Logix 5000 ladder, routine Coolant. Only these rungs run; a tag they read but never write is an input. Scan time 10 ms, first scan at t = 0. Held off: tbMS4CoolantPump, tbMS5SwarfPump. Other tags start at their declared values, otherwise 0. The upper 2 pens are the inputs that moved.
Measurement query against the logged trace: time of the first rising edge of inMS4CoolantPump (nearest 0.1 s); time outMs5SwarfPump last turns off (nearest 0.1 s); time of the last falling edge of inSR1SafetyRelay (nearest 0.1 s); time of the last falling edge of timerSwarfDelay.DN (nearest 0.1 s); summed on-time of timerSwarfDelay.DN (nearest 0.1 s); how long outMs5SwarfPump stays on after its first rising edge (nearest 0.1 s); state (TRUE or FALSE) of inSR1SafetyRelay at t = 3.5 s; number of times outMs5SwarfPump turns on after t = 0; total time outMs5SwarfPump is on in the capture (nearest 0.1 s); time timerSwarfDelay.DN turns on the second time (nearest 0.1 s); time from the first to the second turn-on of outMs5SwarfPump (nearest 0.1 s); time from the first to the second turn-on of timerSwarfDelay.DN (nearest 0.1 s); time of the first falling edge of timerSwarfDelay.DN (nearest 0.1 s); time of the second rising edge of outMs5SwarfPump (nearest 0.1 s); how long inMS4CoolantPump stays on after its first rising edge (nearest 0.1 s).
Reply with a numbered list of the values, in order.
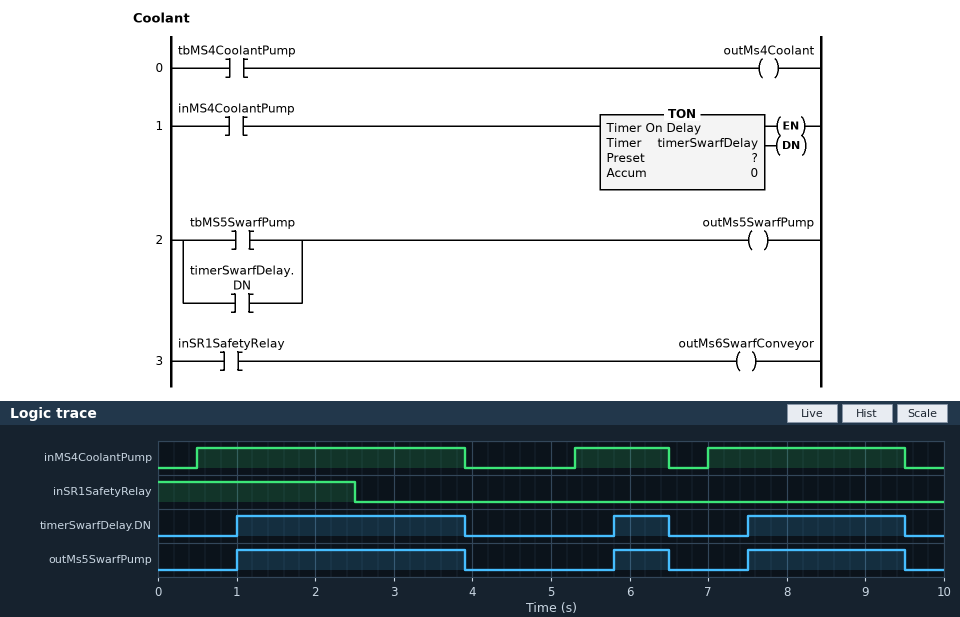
1. 0.5 s
2. 9.5 s
3. 2.5 s
4. 9.5 s
5. 5.6 s
6. 2.9 s
7. FALSE
8. 3
9. 5.6 s
10. 5.8 s
11. 4.8 s
12. 4.8 s
13. 3.9 s
14. 5.8 s
15. 3.4 s
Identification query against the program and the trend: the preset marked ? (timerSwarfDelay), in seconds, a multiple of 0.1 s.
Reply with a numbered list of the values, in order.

1. 0.5 s
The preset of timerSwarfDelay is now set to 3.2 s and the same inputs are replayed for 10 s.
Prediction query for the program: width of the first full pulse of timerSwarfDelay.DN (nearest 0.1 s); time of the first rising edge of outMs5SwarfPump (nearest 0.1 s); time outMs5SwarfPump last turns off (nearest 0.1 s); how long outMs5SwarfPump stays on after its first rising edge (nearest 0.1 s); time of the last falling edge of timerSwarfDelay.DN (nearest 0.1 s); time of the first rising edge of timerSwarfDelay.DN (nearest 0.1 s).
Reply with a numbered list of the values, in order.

1. 0.2 s
2. 3.7 s
3. 3.9 s
4. 0.2 s
5. 3.9 s
6. 3.7 s
